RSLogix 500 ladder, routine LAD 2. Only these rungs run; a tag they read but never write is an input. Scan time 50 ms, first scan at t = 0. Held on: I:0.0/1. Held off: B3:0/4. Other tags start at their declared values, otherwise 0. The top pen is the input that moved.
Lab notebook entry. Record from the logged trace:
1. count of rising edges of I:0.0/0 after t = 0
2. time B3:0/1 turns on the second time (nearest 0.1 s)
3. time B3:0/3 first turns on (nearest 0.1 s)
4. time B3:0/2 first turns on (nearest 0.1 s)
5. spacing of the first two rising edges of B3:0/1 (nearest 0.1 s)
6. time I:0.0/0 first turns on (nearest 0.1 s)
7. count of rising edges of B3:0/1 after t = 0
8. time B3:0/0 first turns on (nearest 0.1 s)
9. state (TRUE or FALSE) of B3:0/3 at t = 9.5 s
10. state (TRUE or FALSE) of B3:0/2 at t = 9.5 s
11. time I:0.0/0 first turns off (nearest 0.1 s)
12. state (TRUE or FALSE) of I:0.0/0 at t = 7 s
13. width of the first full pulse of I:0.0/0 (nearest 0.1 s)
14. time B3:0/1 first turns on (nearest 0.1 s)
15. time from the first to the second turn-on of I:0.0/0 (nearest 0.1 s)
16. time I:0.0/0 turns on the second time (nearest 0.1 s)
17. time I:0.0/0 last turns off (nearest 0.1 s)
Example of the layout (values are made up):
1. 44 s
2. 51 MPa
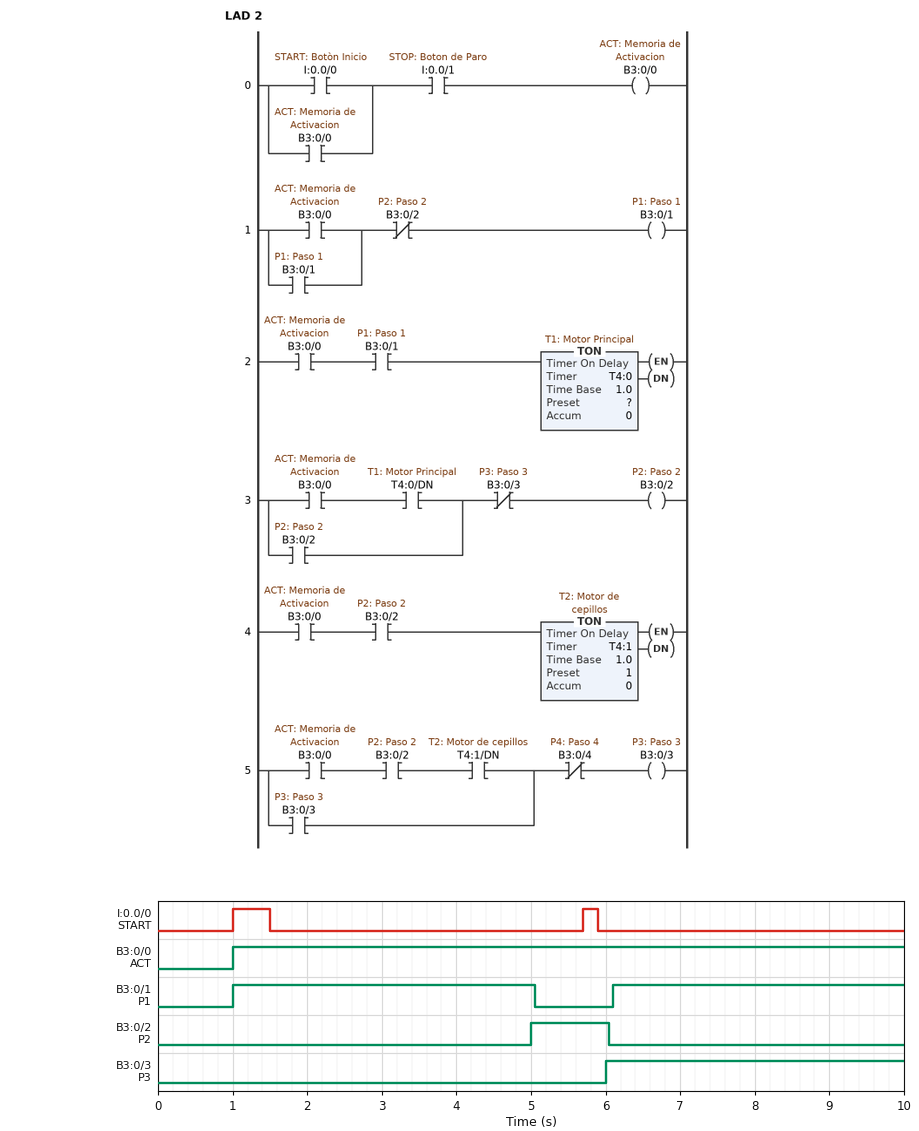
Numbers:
1. 2
2. 6.1 s
3. 6.0 s
4. 5.0 s
5. 5.1 s
6. 1.0 s
7. 2
8. 1.0 s
9. TRUE
10. FALSE
11. 1.5 s
12. FALSE
13. 0.5 s
14. 1.0 s
15. 4.7 s
16. 5.7 s
17. 5.9 s
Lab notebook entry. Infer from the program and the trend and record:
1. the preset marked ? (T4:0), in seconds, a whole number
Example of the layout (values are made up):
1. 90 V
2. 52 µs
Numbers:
1. 4 s
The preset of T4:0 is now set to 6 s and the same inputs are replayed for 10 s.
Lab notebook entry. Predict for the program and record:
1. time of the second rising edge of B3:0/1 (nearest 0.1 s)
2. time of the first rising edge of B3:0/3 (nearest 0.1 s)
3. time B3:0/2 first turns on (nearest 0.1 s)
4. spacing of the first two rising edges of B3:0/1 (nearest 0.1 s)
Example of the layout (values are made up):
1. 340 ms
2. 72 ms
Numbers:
1. 8.1 s
2. 8.0 s
3. 7.0 s
4. 7.1 s
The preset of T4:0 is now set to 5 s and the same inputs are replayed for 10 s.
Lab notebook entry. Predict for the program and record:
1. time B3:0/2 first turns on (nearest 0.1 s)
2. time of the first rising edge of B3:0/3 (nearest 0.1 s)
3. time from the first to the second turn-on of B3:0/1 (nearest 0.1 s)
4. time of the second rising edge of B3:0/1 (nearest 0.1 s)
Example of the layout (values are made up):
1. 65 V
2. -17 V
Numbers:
1. 6.0 s
2. 7.0 s
3. 6.1 s
4. 7.1 s
